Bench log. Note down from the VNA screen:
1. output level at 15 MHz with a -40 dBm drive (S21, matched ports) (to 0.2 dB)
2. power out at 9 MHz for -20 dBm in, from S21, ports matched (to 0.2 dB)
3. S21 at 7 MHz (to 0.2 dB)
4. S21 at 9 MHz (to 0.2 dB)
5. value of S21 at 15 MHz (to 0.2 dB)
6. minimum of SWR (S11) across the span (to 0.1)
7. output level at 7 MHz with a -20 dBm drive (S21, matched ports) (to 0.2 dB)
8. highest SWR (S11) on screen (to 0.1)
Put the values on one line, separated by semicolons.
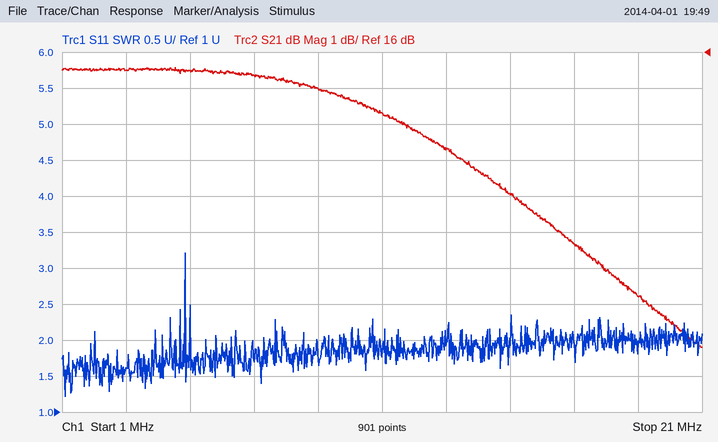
-28.0 dBm; -5.0 dBm; 15.4 dB; 15.0 dB; 12.0 dB; 1.2; -4.6 dBm; 3.2
